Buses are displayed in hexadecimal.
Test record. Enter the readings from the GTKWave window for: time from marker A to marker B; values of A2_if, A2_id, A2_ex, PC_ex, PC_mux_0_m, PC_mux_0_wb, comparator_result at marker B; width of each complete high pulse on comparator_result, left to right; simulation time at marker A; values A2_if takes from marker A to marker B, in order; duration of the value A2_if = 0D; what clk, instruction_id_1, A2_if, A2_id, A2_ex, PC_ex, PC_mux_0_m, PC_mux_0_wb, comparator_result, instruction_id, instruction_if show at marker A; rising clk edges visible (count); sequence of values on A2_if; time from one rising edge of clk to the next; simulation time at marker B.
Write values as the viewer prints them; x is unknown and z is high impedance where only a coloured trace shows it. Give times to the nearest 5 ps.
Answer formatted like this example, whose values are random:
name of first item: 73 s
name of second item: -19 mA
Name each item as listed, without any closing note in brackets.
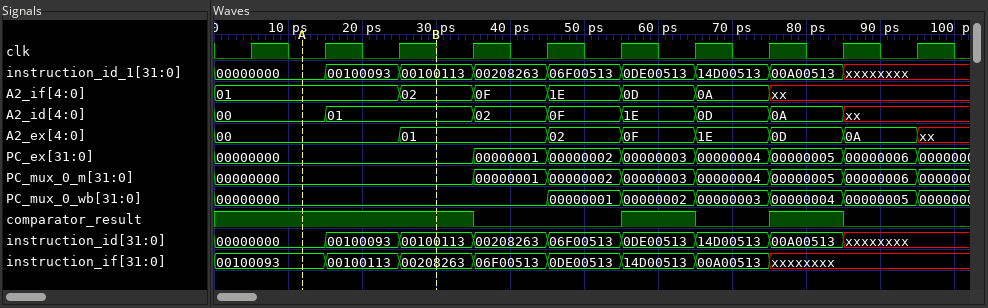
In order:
time from marker A to marker B: 20 ps
values of A2_if, A2_id, A2_ex, PC_ex, PC_mux_0_m, PC_mux_0_wb, comparator_result at marker B: A2_if=02, A2_id=01, A2_ex=01, PC_ex=00000000, PC_mux_0_m=00000000, PC_mux_0_wb=00000000, comparator_result=1
width of each complete high pulse on comparator_result, left to right: 10 ps, 10 ps
simulation time at marker A: 10 ps
values A2_if takes from marker A to marker B, in order: 01, 02
duration of the value A2_if = 0D: 10 ps
what clk, instruction_id_1, A2_if, A2_id, A2_ex, PC_ex, PC_mux_0_m, PC_mux_0_wb, comparator_result, instruction_id, instruction_if show at marker A: clk=0, instruction_id_1=00000000, A2_if=01, A2_id=00, A2_ex=00, PC_ex=00000000, PC_mux_0_m=00000000, PC_mux_0_wb=00000000, comparator_result=1, instruction_id=00000000, instruction_if=00100093
rising clk edges visible: 10
sequence of values on A2_if: 01, 02, 0F, 1E, 0D, 0A, xx
time from one rising edge of clk to the next: 10 ps
simulation time at marker B: 30 ps
